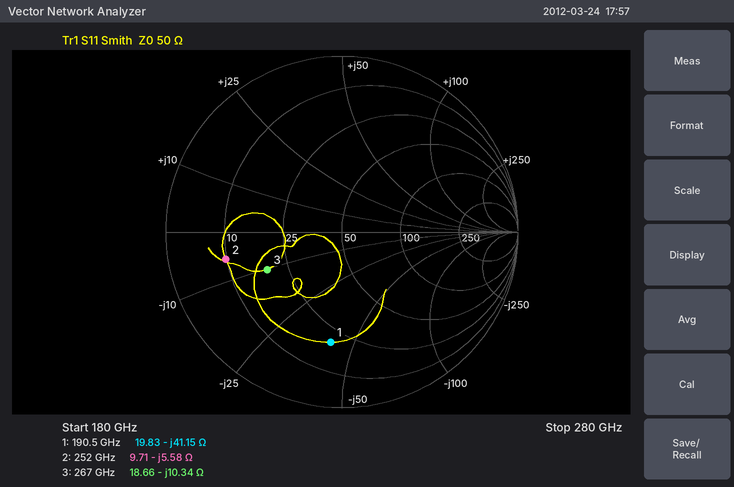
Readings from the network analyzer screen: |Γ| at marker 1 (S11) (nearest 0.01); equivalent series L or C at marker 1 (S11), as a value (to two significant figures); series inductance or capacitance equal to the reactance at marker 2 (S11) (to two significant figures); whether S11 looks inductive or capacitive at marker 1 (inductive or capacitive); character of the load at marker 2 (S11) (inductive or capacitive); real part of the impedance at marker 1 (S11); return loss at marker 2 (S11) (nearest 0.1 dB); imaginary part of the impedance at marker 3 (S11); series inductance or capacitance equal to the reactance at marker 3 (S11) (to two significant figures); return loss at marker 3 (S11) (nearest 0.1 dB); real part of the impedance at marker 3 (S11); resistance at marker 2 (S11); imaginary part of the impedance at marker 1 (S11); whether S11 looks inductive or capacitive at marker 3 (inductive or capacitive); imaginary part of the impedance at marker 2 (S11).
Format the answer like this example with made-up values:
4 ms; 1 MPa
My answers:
0.63; 20 fF; 110 fF; capacitive; capacitive; 19.83 Ω; 3.4 dB; -10.34 Ω; 58 fF; 6.5 dB; 18.66 Ω; 9.71 Ω; -41.15 Ω; capacitive; -5.58 Ω
